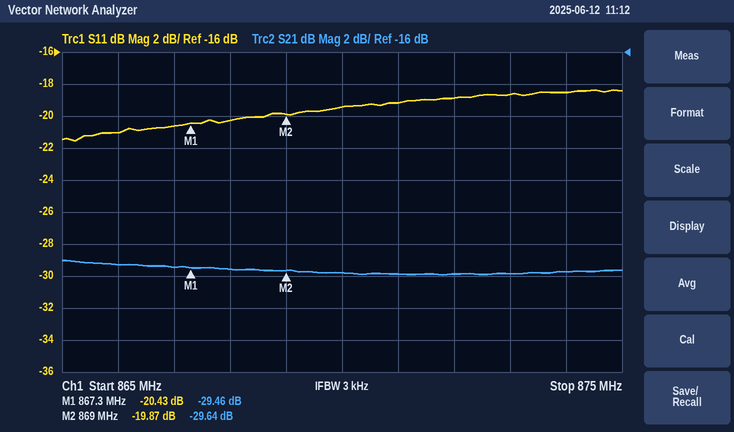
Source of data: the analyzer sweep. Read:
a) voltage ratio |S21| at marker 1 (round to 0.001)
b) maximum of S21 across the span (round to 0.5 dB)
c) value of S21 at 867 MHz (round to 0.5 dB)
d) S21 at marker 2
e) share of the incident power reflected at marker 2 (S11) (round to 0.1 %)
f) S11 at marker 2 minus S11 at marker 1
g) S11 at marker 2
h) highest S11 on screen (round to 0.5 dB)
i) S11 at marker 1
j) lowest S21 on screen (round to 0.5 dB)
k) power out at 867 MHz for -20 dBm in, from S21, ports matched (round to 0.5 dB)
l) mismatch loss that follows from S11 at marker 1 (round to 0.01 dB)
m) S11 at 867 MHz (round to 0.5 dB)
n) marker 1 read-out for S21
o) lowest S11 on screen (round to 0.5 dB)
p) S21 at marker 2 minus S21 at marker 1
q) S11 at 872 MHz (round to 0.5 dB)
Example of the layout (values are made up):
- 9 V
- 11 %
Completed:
- 0.034
- -29.0 dB
- -29.5 dB
- -29.64 dB
- 1.0 %
- 0.56 dB
- -19.87 dB
- -18.5 dB
- -20.43 dB
- -30.0 dB
- -49.5 dBm
- 0.04 dB
- -20.5 dB
- -29.46 dB
- -21.5 dB
- -0.18 dB
- -19.0 dB
